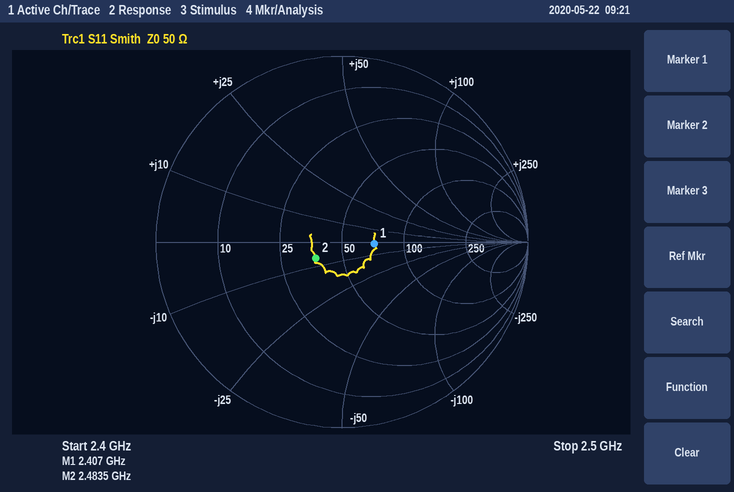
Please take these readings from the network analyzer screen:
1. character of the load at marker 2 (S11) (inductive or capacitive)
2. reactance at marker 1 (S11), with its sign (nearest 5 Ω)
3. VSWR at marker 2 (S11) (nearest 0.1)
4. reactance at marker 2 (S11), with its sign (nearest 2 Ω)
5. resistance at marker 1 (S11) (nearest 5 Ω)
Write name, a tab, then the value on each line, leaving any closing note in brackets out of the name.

character of the load at marker 2 (S11)	capacitive
reactance at marker 1 (S11), with its sign	0 Ω
VSWR at marker 2 (S11)	1.4
reactance at marker 2 (S11), with its sign	-6 Ω
resistance at marker 1 (S11)	70 Ω
